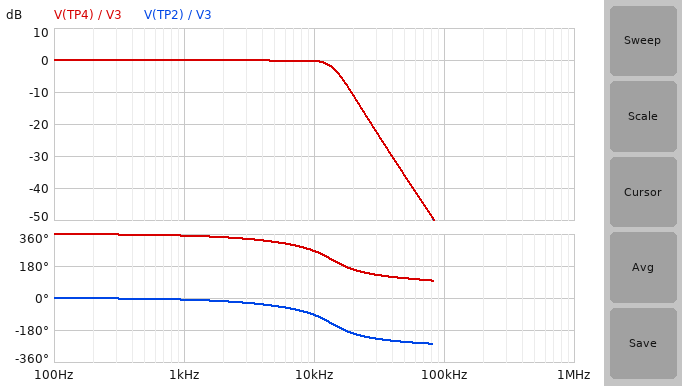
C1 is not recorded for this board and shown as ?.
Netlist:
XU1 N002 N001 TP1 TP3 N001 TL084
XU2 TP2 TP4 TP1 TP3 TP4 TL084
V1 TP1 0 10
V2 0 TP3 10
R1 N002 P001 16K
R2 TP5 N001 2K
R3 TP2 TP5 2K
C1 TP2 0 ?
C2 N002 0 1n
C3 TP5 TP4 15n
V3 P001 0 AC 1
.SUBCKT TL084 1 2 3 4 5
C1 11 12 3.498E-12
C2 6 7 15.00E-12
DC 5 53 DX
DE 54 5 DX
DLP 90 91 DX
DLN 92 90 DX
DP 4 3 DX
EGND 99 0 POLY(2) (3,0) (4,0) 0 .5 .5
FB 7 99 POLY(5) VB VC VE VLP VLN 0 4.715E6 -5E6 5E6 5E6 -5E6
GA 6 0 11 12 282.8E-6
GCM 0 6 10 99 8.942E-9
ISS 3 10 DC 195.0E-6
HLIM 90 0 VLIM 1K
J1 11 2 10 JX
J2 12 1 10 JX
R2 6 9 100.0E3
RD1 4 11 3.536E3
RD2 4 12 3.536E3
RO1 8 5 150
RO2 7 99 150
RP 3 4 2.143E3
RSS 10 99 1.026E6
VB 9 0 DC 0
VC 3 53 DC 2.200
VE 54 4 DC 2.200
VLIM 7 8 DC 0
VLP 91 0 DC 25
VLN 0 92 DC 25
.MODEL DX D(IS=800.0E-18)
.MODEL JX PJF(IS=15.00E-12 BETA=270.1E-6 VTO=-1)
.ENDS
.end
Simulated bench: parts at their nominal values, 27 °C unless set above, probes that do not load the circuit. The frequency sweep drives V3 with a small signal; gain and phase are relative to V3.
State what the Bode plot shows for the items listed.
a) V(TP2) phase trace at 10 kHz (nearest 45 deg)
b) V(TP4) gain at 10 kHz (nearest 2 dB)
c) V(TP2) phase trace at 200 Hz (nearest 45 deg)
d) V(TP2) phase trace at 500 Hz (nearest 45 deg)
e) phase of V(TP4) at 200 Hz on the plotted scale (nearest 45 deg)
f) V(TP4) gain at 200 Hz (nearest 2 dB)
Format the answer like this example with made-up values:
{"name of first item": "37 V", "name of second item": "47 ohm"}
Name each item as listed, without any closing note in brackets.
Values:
{"V(TP2) phase trace at 10 kHz": "-90 deg", "V(TP4) gain at 10 kHz": "0 dB", "V(TP2) phase trace at 200 Hz": "0 deg", "V(TP2) phase trace at 500 Hz": "0 deg", "phase of V(TP4) at 200 Hz on the plotted scale": "360 deg", "V(TP4) gain at 200 Hz": "0 dB"}
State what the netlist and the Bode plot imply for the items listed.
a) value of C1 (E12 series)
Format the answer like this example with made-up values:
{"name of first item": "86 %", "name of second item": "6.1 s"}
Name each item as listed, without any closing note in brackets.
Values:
{"value of C1": "2.2 nF"}
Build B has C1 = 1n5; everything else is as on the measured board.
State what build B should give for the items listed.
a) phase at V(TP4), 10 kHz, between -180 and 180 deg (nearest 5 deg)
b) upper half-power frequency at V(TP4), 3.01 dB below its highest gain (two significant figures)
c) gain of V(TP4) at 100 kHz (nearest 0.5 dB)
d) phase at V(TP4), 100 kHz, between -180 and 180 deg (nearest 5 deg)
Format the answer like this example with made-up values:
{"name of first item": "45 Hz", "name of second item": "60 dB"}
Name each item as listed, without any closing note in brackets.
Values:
{"phase at V(TP4), 10 kHz, between -180 and 180 deg": "-75 deg", "upper half-power frequency at V(TP4), 3.01 dB below its highest gain": "18 kHz", "gain of V(TP4) at 100 kHz": "-51.5 dB", "phase at V(TP4), 100 kHz, between -180 and 180 deg": "95 deg"}
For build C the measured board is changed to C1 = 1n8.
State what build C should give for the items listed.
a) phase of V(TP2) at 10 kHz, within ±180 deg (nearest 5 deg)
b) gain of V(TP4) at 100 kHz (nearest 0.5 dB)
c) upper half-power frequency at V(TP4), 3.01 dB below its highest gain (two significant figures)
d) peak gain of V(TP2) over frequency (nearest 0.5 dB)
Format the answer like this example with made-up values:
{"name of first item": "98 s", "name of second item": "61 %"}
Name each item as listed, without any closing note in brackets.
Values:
{"phase of V(TP2) at 10 kHz, within ±180 deg": "-85 deg", "gain of V(TP4) at 100 kHz": "-53.0 dB", "upper half-power frequency at V(TP4), 3.01 dB below its highest gain": "16 kHz", "peak gain of V(TP2) over frequency": "0 dB"}
